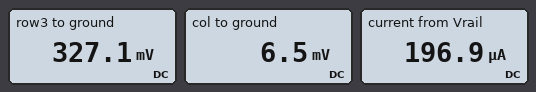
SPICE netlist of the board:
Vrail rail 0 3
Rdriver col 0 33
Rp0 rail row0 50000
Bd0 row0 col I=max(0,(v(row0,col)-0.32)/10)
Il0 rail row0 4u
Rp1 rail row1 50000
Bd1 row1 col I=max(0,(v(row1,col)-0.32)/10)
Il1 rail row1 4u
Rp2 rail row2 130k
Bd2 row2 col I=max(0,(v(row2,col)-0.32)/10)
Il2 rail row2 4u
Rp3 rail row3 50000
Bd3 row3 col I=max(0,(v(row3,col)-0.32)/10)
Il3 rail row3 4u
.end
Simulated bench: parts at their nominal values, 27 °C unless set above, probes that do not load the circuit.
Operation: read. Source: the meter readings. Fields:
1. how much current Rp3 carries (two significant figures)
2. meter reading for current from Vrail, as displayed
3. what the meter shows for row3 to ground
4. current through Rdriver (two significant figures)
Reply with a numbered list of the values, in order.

1. 53 µA
2. 196.9 µA
3. 327.1 mV
4. 200 µA
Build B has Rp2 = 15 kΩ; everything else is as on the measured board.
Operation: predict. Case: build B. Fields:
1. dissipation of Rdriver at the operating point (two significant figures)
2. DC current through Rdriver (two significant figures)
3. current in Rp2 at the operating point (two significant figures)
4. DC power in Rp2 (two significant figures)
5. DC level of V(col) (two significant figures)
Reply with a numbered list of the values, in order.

1. 4.1 µW
2. 350 µA
3. 180 µA
4. 470 µW
5. 12 mV
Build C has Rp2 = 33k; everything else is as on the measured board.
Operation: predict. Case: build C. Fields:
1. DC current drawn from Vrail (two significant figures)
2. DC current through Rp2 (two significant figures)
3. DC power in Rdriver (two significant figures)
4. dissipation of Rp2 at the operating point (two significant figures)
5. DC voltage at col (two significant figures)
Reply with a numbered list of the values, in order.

1. 260 µA
2. 81 µA
3. 2.2 µW
4. 220 µW
5. 8.5 mV
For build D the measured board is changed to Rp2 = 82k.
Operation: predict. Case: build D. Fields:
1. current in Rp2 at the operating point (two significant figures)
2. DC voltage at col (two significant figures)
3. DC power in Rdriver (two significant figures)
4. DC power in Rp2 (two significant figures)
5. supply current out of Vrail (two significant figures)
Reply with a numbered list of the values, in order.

1. 33 µA
2. 6.9 mV
3. 1.4 µW
4. 87 µW
5. 210 µA
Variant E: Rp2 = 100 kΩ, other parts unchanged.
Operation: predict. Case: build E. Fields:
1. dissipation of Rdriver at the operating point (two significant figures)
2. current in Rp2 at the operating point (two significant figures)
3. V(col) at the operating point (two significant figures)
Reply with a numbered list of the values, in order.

1. 1.4 µW
2. 27 µA
3. 6.7 mV
